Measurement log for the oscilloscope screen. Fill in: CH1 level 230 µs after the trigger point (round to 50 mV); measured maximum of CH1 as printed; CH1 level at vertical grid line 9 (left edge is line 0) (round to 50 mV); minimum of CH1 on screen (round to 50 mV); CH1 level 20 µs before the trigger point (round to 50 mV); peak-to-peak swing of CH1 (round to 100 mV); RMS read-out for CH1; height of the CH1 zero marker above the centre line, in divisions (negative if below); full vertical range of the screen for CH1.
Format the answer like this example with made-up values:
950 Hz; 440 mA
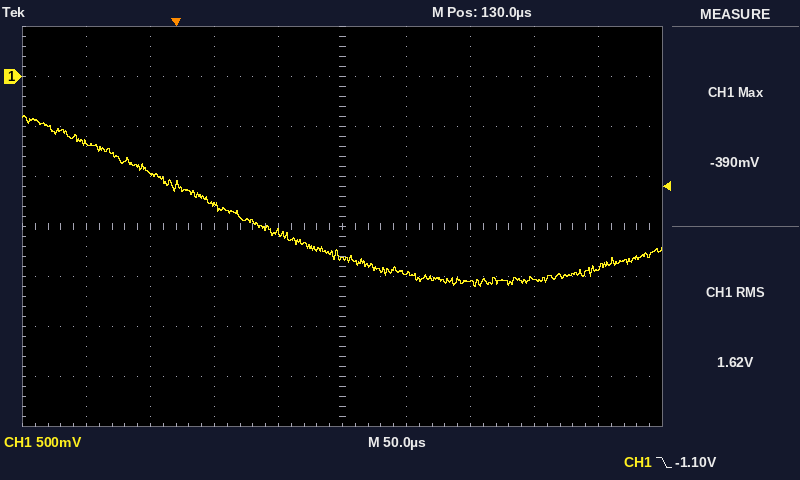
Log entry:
-2.05 V; -390 mV; -1.90 V; -2.10 V; -950 mV; 1.70 V; 1.62 V; +3.0 div; 4 V
